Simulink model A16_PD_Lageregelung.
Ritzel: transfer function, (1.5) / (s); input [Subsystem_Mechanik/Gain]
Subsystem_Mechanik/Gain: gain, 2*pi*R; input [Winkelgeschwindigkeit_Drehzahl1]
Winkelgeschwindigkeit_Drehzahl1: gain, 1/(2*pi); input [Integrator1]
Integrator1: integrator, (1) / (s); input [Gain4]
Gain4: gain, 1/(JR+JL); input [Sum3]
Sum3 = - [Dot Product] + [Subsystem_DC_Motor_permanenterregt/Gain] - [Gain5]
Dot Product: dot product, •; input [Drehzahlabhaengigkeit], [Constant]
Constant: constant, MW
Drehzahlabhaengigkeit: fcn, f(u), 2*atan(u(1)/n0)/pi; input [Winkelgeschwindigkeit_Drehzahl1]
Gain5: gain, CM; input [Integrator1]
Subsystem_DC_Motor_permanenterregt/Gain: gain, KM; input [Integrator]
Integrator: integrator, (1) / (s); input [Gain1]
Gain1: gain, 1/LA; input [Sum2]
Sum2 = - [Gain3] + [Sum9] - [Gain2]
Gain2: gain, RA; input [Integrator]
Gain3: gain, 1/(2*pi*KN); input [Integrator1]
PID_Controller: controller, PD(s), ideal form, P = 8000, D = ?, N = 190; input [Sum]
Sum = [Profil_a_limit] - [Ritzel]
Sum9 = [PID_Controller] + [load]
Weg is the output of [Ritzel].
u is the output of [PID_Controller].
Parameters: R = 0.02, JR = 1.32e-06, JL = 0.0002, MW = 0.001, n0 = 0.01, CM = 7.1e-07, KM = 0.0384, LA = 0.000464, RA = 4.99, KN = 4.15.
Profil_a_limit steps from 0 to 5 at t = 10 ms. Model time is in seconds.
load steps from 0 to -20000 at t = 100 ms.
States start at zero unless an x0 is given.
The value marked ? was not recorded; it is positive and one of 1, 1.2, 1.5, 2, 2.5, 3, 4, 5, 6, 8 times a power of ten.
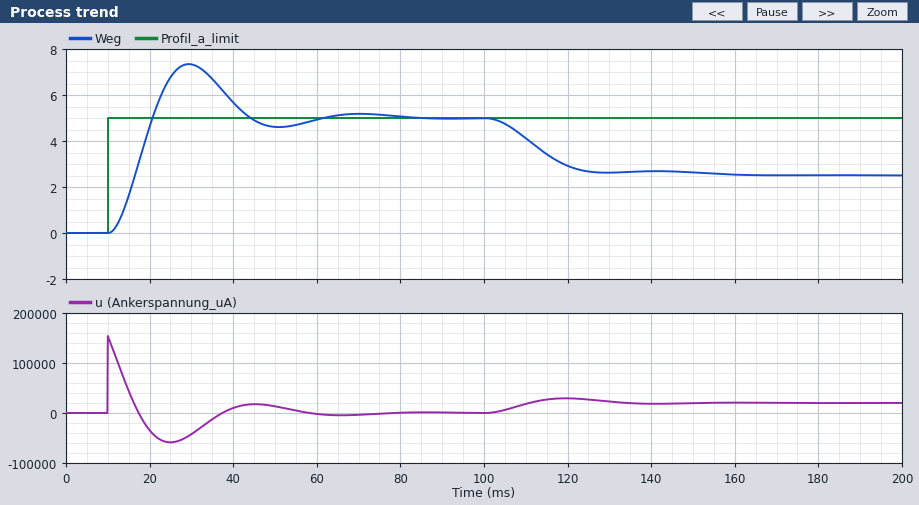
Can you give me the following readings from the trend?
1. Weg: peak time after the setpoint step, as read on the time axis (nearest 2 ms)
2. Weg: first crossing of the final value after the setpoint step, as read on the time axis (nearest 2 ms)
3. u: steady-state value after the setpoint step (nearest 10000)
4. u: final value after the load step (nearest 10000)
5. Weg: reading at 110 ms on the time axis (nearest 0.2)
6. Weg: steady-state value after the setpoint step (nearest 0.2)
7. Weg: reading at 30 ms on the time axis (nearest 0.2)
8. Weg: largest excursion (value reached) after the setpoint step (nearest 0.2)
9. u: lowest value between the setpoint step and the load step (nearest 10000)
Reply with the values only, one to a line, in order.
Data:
30 ms
20 ms
0
20000
4.2
5.0
7.4
7.4
-60000
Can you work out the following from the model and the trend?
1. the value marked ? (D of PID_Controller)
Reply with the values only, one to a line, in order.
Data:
0.015
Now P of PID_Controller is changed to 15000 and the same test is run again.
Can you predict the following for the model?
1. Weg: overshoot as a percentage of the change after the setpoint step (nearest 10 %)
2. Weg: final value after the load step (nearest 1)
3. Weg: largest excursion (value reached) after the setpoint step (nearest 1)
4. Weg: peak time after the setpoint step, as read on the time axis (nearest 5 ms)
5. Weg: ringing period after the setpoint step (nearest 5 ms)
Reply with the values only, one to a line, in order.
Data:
50 %
4
8
25 ms
25 ms
